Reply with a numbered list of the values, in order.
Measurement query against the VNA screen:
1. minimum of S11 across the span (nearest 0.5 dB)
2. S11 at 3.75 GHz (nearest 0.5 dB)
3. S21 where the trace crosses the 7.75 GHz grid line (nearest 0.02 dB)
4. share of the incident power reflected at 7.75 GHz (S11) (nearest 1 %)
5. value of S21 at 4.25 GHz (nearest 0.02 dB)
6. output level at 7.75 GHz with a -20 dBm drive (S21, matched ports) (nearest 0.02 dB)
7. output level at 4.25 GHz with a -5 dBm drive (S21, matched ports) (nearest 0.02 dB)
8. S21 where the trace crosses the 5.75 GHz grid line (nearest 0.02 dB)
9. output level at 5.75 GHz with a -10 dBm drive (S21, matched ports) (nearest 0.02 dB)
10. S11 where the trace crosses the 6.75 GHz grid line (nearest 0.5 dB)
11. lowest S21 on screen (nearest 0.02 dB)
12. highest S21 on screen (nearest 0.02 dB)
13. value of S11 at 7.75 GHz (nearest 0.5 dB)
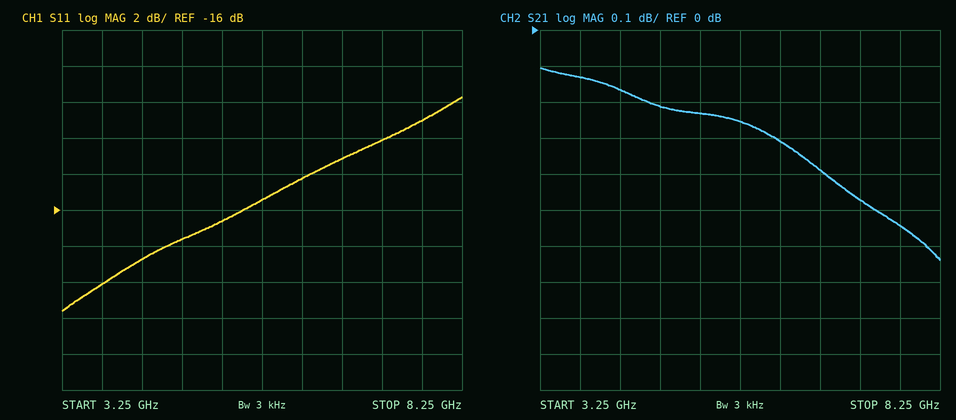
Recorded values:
1. -21.5 dB
2. -20.0 dB
3. -0.54 dB
4. 8 %
5. -0.16 dB
6. -20.54 dBm
7. -5.16 dBm
8. -0.26 dB
9. -10.26 dBm
10. -13.0 dB
11. -0.64 dB
12. -0.10 dB
13. -11.0 dB
